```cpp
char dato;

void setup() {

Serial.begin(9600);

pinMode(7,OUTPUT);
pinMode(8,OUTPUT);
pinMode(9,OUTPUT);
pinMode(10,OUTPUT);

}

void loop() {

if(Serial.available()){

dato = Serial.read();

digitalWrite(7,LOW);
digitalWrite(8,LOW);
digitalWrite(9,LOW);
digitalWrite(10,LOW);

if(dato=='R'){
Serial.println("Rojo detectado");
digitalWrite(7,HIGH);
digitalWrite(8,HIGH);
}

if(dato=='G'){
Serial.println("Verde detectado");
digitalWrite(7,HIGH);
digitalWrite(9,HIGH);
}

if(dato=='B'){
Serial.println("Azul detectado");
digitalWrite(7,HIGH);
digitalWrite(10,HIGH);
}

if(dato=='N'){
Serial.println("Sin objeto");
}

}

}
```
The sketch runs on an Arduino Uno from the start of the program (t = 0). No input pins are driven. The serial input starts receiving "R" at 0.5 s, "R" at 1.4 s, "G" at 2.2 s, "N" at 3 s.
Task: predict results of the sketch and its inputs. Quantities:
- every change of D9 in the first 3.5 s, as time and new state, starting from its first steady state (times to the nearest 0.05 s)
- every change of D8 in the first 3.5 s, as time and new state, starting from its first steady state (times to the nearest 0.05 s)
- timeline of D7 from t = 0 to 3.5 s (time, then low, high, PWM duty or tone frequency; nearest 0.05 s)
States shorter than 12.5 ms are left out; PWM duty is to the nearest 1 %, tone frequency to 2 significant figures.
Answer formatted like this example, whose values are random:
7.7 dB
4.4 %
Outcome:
0 s low; 2.2 s high; 3 s low
0 s low; 0.5 s high; 2.2 s low
0 s low; 0.5 s high; 3 s low
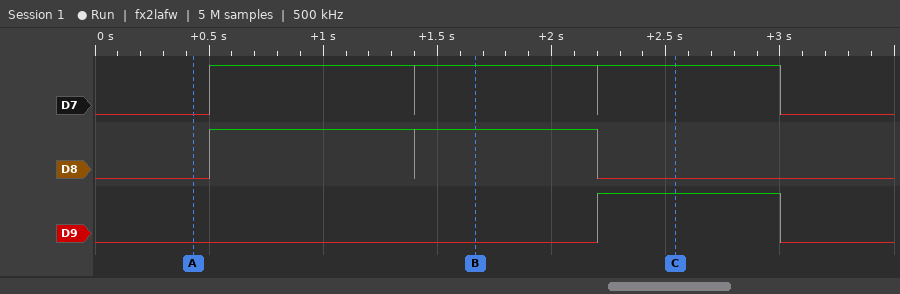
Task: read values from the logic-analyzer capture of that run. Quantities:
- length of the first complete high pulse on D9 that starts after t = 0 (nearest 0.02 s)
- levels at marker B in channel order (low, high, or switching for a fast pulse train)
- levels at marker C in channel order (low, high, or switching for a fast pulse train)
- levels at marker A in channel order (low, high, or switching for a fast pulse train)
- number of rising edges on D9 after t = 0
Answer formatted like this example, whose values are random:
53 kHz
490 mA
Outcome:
0.80 s
D7 high, D8 high, D9 low
D7 high, D8 low, D9 high
D7 low, D8 low, D9 low
1
